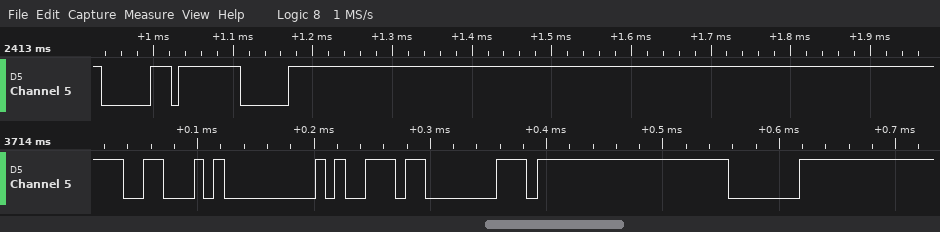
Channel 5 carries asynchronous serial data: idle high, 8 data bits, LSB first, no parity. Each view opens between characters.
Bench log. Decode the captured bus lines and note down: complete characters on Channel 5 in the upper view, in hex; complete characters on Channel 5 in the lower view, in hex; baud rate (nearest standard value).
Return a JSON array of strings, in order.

["C0, FF, C0", "46, 00, B9, C0, FF, C0", "115200 baud"]
